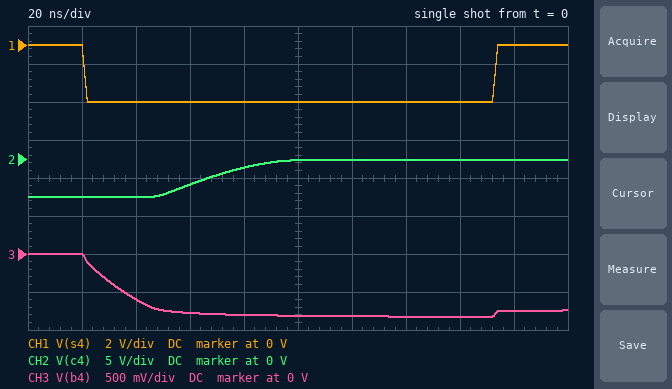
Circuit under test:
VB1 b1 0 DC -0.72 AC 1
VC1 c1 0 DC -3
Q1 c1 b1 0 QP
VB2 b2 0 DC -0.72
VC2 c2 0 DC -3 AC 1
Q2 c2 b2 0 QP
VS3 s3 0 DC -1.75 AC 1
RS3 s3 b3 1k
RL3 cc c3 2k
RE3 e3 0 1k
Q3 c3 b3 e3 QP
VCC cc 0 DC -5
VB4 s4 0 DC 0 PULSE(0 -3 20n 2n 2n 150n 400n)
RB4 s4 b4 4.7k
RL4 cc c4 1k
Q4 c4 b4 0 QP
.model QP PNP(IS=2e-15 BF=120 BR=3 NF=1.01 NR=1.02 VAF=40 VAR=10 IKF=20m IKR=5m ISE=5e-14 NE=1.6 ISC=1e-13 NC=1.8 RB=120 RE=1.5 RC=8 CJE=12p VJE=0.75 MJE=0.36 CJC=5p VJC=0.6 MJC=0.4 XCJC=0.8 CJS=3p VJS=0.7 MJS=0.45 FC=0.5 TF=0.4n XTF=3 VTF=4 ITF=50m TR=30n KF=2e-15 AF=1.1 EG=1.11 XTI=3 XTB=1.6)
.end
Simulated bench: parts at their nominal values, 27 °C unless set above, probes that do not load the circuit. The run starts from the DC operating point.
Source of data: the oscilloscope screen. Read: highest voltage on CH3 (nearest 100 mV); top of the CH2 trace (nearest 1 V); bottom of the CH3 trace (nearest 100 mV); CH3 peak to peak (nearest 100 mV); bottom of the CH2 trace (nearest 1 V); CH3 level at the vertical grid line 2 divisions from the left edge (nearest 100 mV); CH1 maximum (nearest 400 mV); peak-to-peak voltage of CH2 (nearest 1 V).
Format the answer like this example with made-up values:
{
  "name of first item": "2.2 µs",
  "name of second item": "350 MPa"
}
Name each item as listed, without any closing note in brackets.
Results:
{
  "highest voltage on CH3": "0 V",
  "top of the CH2 trace": "0 V",
  "bottom of the CH3 trace": "-800 mV",
  "CH3 peak to peak": "800 mV",
  "bottom of the CH2 trace": "-5 V",
  "CH3 level at the vertical grid line 2 divisions from the left edge": "-600 mV",
  "CH1 maximum": "0 V",
  "peak-to-peak voltage of CH2": "5 V"
}
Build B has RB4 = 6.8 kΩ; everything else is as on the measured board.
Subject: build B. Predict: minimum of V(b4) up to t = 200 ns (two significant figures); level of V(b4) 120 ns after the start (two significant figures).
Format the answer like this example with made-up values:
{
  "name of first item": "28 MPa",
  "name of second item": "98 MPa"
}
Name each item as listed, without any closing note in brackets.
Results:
{
  "minimum of V(b4) up to t = 200 ns": "-800 mV",
  "level of V(b4) 120 ns after the start": "-790 mV"
}
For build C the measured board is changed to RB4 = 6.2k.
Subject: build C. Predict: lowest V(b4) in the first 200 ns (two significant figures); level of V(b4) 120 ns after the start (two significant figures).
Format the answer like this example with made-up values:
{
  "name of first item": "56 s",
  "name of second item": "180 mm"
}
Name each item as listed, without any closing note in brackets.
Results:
{
  "lowest V(b4) in the first 200 ns": "-810 mV",
  "level of V(b4) 120 ns after the start": "-800 mV"
}
